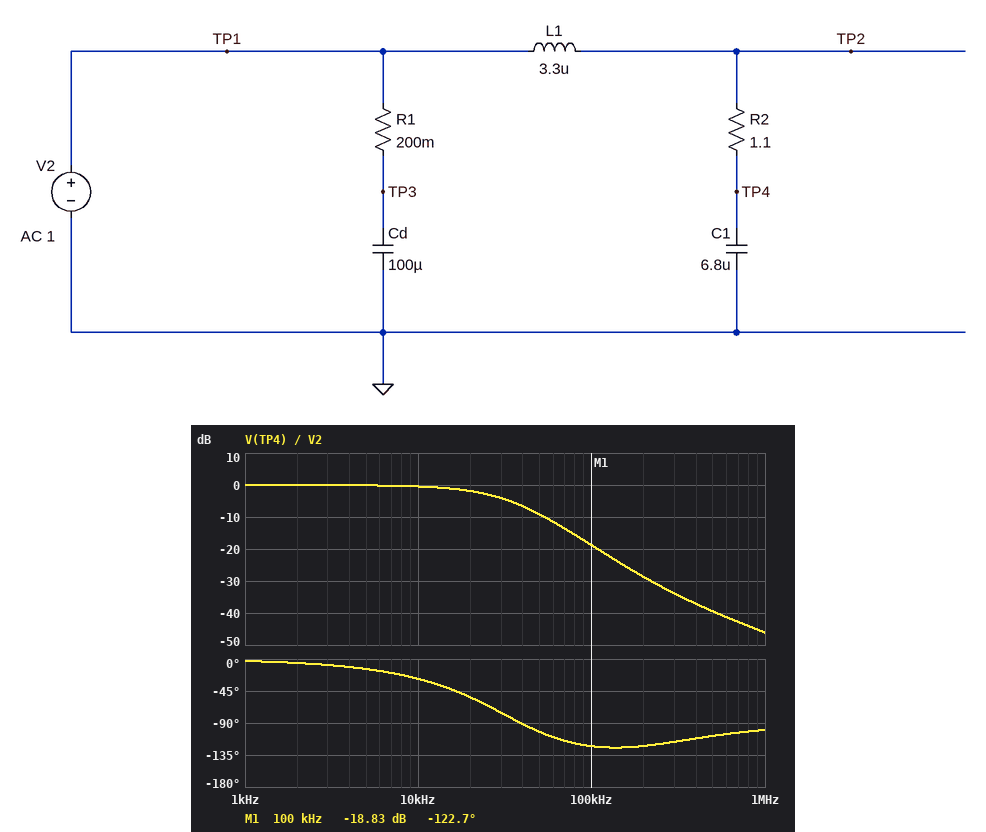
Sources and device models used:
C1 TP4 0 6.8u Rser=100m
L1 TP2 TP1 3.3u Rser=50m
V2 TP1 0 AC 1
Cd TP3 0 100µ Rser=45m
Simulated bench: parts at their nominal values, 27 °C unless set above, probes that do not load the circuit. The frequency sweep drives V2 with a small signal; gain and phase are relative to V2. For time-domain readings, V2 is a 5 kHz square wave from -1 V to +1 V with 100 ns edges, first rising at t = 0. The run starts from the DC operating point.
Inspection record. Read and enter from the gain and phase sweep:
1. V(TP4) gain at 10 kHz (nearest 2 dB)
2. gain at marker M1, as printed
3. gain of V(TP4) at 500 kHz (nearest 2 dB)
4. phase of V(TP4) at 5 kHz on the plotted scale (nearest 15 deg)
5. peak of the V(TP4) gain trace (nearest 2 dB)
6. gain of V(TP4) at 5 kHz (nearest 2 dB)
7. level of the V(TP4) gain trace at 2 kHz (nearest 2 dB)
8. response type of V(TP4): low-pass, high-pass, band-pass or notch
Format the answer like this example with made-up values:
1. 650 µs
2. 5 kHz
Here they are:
1. 0 dB
2. -18.83 dB
3. -40 dB
4. -15 deg
5. 0 dB
6. 0 dB
7. 0 dB
8. low-pass
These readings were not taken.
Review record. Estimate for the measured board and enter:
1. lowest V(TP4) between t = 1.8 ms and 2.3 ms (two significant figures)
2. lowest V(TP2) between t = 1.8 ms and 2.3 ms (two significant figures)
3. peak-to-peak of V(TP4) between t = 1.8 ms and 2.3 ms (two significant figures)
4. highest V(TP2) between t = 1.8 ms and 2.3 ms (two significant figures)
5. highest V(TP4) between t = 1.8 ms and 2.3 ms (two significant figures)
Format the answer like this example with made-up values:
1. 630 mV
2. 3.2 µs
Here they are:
1. -1.0 V
2. -1.3 V
3. 2.0 V
4. 1.3 V
5. 1.0 V
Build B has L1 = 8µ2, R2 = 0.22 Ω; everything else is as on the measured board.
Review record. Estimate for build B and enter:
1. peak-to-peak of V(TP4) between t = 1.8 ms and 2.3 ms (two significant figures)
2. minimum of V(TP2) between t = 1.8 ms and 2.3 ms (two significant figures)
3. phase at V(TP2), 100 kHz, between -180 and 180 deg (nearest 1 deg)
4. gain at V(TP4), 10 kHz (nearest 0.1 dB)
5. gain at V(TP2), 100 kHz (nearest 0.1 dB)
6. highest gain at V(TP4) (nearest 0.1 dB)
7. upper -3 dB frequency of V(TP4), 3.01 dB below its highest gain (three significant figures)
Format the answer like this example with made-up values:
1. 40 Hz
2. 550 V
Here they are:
1. 4.1 V
2. -2.1 V
3. -122 deg
4. 2.0 dB
5. -21.9 dB
6. 9.6 dB
7. 24.1 kHz
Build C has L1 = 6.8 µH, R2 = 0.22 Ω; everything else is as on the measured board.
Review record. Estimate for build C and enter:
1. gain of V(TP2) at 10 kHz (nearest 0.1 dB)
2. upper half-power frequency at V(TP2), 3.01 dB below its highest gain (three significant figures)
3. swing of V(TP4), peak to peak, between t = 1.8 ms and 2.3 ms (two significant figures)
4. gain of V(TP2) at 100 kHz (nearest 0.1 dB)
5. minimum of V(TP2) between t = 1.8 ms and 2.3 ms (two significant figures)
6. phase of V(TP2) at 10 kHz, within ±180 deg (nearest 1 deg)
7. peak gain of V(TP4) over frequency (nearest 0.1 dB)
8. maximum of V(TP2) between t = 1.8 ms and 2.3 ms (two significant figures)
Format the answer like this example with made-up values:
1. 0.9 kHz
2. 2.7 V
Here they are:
1. 1.7 dB
2. 26.8 kHz
3. 4.2 V
4. -20.2 dB
5. -2.2 V
6. -3 deg
7. 8.8 dB
8. 2.2 V
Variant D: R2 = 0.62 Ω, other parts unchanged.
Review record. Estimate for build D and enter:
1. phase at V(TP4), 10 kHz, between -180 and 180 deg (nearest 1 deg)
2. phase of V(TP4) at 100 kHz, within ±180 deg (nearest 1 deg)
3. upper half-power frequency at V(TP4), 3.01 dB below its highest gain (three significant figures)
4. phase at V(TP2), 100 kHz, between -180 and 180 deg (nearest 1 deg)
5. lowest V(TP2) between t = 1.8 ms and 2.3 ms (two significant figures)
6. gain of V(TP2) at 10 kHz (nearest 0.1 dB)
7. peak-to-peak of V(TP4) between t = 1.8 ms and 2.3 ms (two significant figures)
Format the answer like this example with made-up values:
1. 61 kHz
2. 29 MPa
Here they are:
1. -17 deg
2. -134 deg
3. 38.7 kHz
4. -85 deg
5. -1.5 V
6. 0.7 dB
7. 2.5 V
